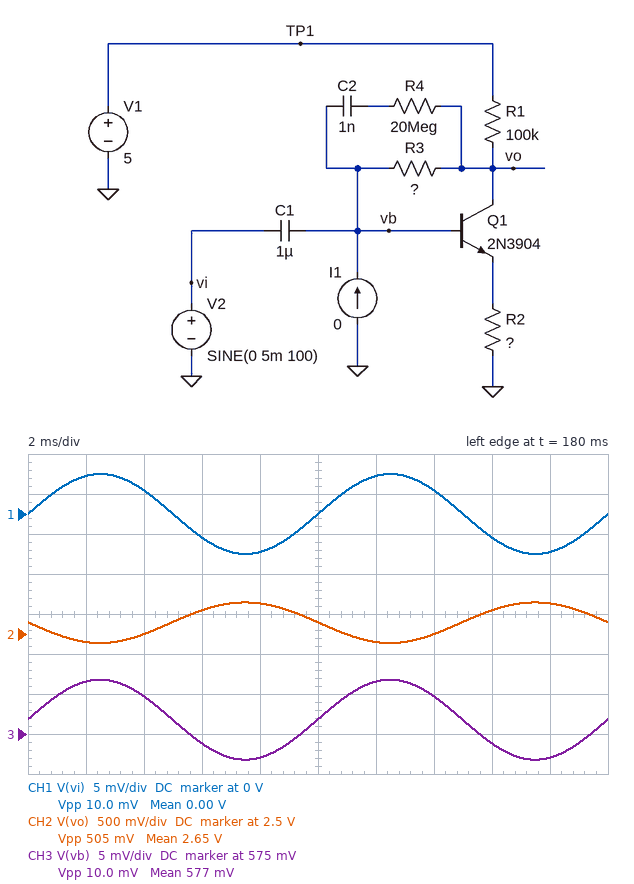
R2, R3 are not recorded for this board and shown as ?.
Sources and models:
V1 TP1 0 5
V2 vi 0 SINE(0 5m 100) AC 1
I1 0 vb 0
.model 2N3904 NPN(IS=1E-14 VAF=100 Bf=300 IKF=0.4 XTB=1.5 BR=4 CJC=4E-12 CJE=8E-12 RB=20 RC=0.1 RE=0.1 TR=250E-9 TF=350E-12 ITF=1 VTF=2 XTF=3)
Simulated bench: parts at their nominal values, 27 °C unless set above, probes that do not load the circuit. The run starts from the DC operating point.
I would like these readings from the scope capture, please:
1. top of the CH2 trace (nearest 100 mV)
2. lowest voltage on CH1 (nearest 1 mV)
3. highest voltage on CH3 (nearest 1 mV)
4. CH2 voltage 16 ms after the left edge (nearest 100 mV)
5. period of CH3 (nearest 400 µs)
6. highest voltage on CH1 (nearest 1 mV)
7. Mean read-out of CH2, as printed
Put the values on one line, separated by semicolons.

2.9 V; -5 mV; 582 mV; 2.8 V; 10.0 ms; 5 mV; 2.65 V
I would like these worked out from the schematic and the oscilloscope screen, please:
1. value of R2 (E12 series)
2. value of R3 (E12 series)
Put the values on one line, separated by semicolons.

820 Ω; 27 MΩ
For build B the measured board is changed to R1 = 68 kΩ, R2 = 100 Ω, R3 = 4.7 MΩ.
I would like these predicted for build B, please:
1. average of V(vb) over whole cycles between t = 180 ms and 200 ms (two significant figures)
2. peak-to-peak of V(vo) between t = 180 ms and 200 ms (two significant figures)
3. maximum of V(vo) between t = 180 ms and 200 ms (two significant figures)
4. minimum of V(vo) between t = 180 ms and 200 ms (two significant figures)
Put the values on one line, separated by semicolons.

580 mV; 1.1 V; 1.9 V; 840 mV
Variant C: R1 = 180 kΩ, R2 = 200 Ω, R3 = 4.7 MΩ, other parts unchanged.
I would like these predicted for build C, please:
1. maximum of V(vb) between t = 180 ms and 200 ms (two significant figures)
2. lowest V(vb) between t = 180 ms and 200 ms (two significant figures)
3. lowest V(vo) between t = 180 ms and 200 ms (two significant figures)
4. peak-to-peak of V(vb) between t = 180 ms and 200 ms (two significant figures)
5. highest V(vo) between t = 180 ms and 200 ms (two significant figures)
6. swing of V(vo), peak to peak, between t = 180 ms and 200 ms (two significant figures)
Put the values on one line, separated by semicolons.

570 mV; 560 mV; 280 mV; 10 mV; 1.5 V; 1.2 V
